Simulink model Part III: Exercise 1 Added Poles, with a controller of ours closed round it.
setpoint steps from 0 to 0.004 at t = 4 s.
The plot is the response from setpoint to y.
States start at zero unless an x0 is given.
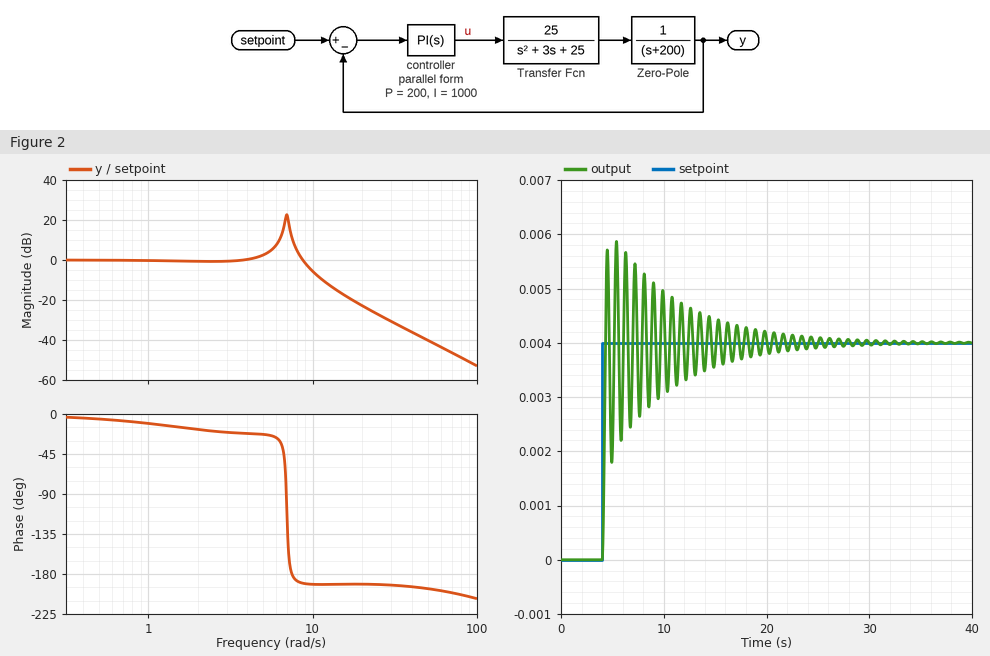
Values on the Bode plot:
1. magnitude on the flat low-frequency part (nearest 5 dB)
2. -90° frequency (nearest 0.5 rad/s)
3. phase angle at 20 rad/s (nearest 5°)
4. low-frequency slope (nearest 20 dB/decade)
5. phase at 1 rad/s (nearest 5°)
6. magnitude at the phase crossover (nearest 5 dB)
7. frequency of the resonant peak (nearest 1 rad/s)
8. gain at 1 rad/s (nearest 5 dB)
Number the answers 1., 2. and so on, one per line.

1. 0 dB
2. 7.0 rad/s
3. -190°
4. 0 dB/decade
5. -10°
6. 10 dB
7. 7 rad/s
8. 0 dB
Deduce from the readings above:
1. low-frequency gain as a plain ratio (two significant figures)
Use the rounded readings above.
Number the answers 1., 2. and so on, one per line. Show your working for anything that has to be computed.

1. 10^(0 / 20) = 1.0
